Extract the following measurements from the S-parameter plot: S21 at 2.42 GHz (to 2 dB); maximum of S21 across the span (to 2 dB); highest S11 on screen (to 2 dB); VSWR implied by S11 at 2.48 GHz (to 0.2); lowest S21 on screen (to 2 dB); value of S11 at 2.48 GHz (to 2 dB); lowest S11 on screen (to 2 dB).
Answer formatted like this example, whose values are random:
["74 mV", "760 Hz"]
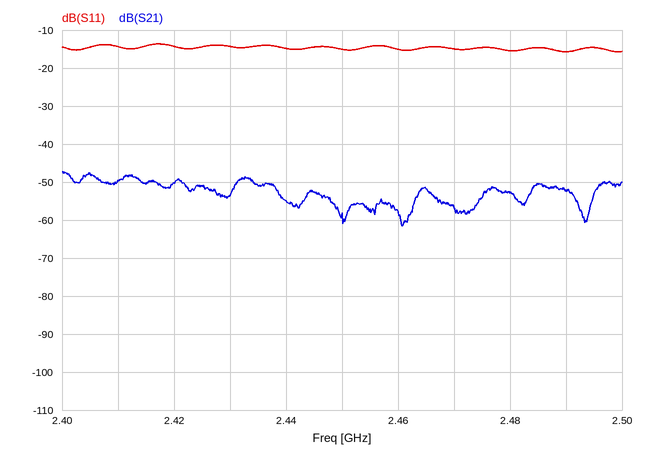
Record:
["-50 dB", "-48 dB", "-14 dB", "1.4", "-62 dB", "-16 dB", "-16 dB"]
